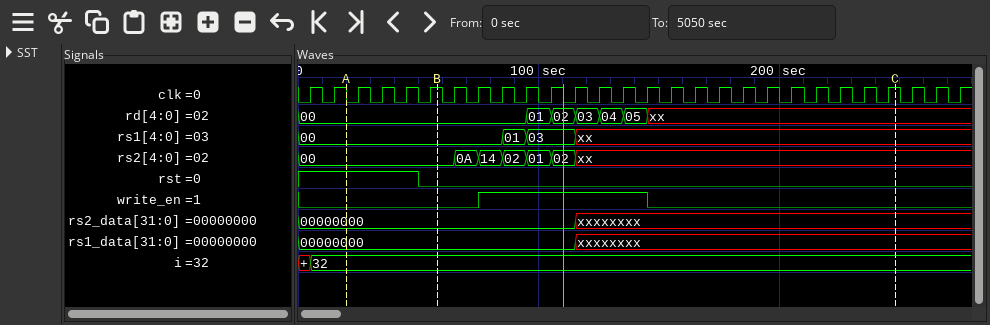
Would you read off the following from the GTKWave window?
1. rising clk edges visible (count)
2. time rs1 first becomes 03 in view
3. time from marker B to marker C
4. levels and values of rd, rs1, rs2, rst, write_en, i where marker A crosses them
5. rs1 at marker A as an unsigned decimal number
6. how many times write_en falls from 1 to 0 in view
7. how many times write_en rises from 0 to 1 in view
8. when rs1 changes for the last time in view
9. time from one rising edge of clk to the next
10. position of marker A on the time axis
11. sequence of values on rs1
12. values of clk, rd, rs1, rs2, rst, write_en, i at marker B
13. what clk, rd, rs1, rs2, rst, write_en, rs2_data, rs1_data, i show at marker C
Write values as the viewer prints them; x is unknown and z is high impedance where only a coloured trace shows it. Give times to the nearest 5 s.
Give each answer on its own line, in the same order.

28
95 s
190 s
rd=00, rs1=00, rs2=00, rst=1, write_en=0, i=32
0
1
1
115 s
10 s
20 s
00, 01, 03, xx
clk=1, rd=00, rs1=00, rs2=00, rst=0, write_en=0, i=32
clk=1, rd=xx, rs1=xx, rs2=xx, rst=0, write_en=0, rs2_data=xxxxxxxx, rs1_data=xxxxxxxx, i=32
